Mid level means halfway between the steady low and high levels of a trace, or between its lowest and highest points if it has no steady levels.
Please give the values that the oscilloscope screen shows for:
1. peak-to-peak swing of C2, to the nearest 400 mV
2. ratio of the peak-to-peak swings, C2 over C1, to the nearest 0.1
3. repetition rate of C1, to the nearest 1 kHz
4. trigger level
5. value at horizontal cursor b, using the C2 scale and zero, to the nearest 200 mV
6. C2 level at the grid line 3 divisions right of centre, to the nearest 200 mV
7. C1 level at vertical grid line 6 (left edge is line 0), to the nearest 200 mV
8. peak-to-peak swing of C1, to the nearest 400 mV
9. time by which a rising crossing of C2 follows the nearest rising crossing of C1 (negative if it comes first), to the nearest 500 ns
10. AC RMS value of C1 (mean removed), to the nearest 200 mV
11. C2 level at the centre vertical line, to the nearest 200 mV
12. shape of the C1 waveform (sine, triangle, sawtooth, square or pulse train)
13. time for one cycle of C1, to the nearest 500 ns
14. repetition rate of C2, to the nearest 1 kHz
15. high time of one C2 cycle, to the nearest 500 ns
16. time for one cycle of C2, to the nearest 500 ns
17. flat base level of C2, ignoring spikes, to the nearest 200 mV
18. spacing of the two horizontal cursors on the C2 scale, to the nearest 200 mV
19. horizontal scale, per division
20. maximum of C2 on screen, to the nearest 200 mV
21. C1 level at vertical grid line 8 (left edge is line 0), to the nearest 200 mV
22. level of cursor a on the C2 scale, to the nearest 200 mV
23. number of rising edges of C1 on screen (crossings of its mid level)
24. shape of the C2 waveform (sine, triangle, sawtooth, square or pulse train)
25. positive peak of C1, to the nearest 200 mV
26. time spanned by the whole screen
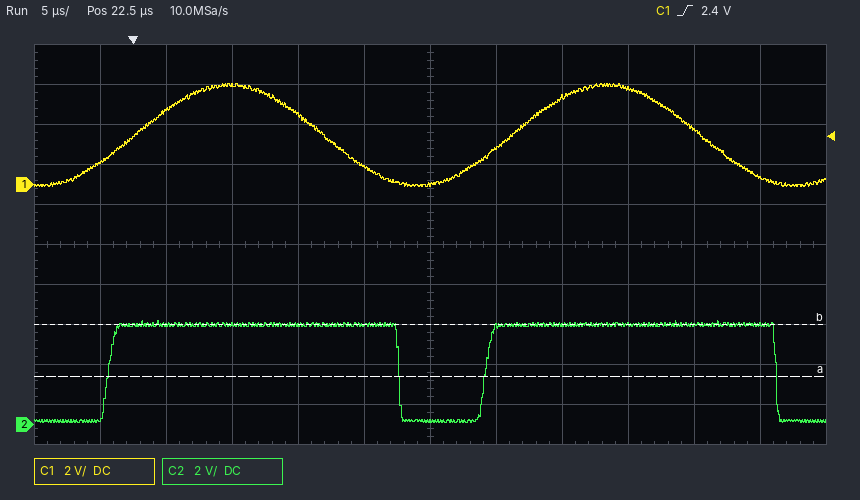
5.2 V
1.0
35 kHz
2.4 V
5.0 V
5.0 V
0.0 V
5.2 V
-2.0 µs
1.8 V
200 mV
sine
28.5 µs
35 kHz
22.0 µs
28.5 µs
200 mV
2.6 V
5 µs
5.2 V
4.4 V
2.4 V
2
pulse train
5.0 V
60 µs
